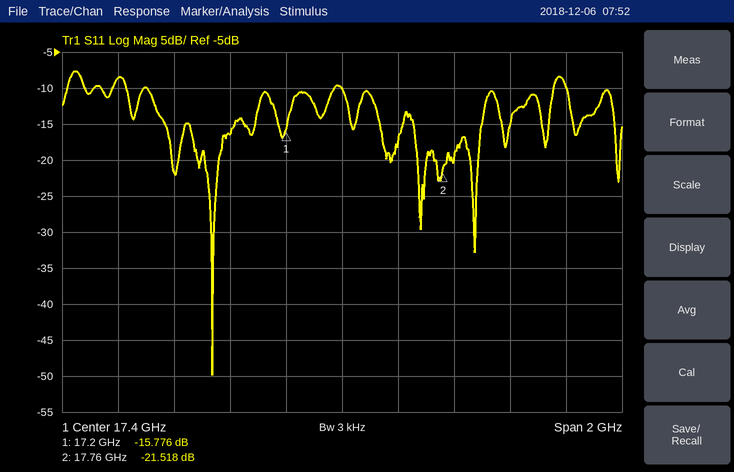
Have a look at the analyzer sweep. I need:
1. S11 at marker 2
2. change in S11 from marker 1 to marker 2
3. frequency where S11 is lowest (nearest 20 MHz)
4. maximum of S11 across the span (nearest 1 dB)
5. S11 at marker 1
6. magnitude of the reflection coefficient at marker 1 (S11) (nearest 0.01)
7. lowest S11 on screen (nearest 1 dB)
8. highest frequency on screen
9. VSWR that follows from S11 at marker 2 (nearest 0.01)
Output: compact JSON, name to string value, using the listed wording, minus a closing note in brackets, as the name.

{"S11 at marker 2": "-21.518 dB", "change in S11 from marker 1 to marker 2": "-5.742 dB", "frequency where S11 is lowest": "16.94 GHz", "maximum of S11 across the span": "-8 dB", "S11 at marker 1": "-15.776 dB", "magnitude of the reflection coefficient at marker 1 (S11)": "0.16", "lowest S11 on screen": "-50 dB", "highest frequency on screen": "18.4 GHz", "VSWR that follows from S11 at marker 2": "1.18"}
